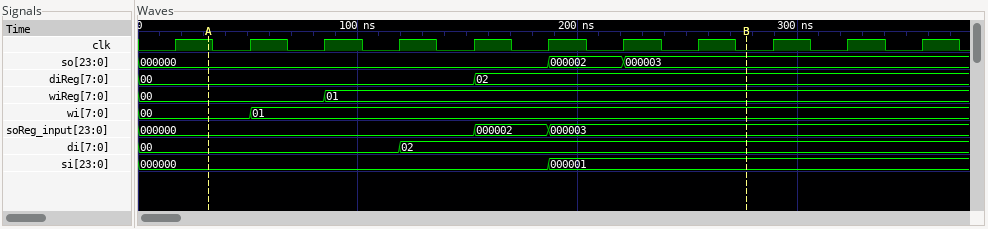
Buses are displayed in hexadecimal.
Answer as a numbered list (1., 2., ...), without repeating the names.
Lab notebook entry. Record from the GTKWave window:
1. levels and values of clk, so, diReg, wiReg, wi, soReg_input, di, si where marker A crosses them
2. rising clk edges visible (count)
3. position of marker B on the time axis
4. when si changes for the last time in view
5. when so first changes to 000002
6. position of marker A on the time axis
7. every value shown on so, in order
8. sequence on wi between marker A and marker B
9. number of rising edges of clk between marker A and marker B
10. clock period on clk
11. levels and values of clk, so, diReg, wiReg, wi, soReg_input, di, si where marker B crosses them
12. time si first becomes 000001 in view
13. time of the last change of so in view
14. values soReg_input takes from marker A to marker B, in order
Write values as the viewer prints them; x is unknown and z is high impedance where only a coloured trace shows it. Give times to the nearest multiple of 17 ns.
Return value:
1. clk=1, so=000000, diReg=00, wiReg=00, wi=00, soReg_input=000000, di=00, si=000000
2. 11
3. 272 ns
4. 187 ns
5. 187 ns
6. 34 ns
7. 000000, 000002, 000003
8. 00, 01
9. 7
10. 34 ns
11. clk=0, so=000003, diReg=02, wiReg=01, wi=01, soReg_input=000003, di=02, si=000001
12. 187 ns
13. 221 ns
14. 000000, 000002, 000003
